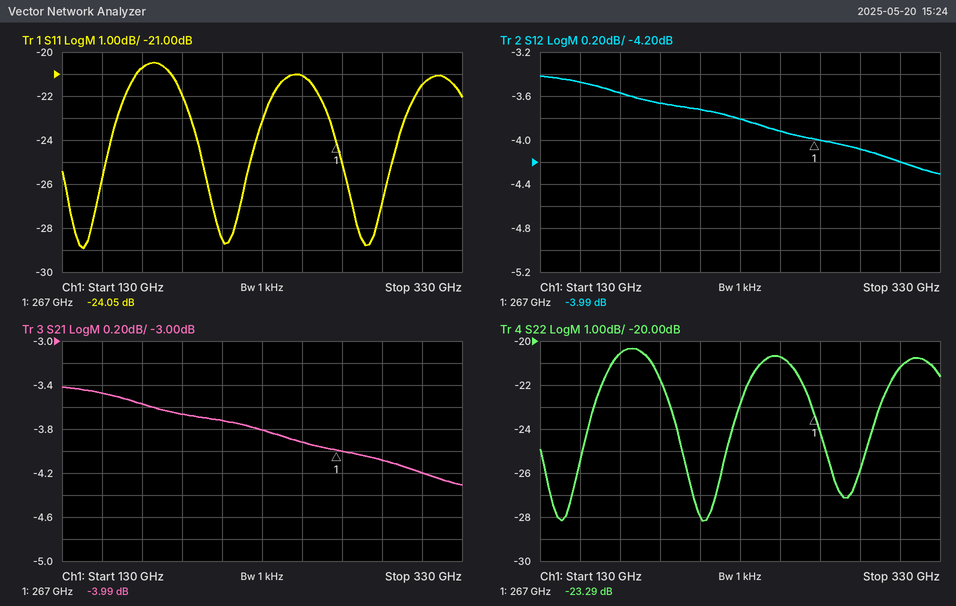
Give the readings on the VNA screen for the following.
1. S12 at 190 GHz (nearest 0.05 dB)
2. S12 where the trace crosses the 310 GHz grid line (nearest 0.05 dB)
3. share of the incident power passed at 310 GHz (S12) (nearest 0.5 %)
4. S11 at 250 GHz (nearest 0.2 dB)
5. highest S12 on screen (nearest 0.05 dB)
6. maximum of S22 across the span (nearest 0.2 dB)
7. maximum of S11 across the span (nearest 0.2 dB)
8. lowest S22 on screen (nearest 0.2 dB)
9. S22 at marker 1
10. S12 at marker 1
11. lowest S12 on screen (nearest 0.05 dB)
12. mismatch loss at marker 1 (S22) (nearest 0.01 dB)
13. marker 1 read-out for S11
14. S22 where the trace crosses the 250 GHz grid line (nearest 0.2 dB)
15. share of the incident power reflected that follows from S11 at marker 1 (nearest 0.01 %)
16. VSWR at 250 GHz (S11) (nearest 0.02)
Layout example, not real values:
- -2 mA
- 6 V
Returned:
- -3.65 dB
- -4.20 dB
- 38.0 %
- -21.0 dB
- -3.40 dB
- -20.4 dB
- -20.4 dB
- -28.2 dB
- -23.29 dB
- -3.99 dB
- -4.30 dB
- 0.02 dB
- -24.05 dB
- -20.8 dB
- 0.39 %
- 1.20
